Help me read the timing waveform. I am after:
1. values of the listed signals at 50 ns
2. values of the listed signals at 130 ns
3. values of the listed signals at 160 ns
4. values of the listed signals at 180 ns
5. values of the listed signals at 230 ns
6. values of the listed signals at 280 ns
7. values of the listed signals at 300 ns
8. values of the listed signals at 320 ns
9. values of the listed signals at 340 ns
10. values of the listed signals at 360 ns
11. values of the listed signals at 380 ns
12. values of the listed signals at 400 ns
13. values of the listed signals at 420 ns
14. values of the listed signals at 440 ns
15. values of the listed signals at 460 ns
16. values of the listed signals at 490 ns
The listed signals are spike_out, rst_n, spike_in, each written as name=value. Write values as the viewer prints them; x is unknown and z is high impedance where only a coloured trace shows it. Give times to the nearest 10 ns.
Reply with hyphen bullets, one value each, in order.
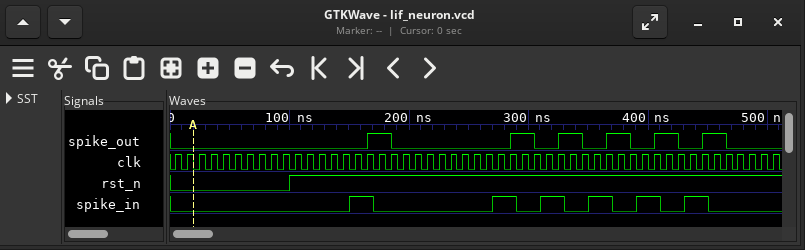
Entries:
- spike_out=0, rst_n=0, spike_in=0
- spike_out=0, rst_n=1, spike_in=0
- spike_out=0, rst_n=1, spike_in=1
- spike_out=1, rst_n=1, spike_in=0
- spike_out=0, rst_n=1, spike_in=0
- spike_out=0, rst_n=1, spike_in=1
- spike_out=1, rst_n=1, spike_in=0
- spike_out=0, rst_n=1, spike_in=1
- spike_out=1, rst_n=1, spike_in=0
- spike_out=0, rst_n=1, spike_in=1
- spike_out=1, rst_n=1, spike_in=0
- spike_out=0, rst_n=1, spike_in=1
- spike_out=1, rst_n=1, spike_in=0
- spike_out=0, rst_n=1, spike_in=1
- spike_out=1, rst_n=1, spike_in=0
- spike_out=0, rst_n=1, spike_in=0
